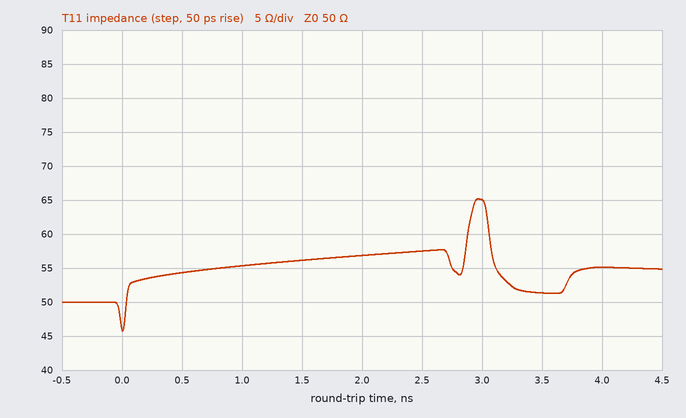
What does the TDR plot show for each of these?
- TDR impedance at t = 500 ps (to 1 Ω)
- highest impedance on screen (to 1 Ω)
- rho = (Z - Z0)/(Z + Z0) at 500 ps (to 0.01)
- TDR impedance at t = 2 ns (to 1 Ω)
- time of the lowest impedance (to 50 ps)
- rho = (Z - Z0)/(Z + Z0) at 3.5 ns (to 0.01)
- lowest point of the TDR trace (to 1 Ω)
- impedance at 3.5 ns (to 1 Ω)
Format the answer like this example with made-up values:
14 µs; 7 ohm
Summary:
54 Ω; 65 Ω; +0.04; 57 Ω; 0 ps; +0.01; 46 Ω; 51 Ω
